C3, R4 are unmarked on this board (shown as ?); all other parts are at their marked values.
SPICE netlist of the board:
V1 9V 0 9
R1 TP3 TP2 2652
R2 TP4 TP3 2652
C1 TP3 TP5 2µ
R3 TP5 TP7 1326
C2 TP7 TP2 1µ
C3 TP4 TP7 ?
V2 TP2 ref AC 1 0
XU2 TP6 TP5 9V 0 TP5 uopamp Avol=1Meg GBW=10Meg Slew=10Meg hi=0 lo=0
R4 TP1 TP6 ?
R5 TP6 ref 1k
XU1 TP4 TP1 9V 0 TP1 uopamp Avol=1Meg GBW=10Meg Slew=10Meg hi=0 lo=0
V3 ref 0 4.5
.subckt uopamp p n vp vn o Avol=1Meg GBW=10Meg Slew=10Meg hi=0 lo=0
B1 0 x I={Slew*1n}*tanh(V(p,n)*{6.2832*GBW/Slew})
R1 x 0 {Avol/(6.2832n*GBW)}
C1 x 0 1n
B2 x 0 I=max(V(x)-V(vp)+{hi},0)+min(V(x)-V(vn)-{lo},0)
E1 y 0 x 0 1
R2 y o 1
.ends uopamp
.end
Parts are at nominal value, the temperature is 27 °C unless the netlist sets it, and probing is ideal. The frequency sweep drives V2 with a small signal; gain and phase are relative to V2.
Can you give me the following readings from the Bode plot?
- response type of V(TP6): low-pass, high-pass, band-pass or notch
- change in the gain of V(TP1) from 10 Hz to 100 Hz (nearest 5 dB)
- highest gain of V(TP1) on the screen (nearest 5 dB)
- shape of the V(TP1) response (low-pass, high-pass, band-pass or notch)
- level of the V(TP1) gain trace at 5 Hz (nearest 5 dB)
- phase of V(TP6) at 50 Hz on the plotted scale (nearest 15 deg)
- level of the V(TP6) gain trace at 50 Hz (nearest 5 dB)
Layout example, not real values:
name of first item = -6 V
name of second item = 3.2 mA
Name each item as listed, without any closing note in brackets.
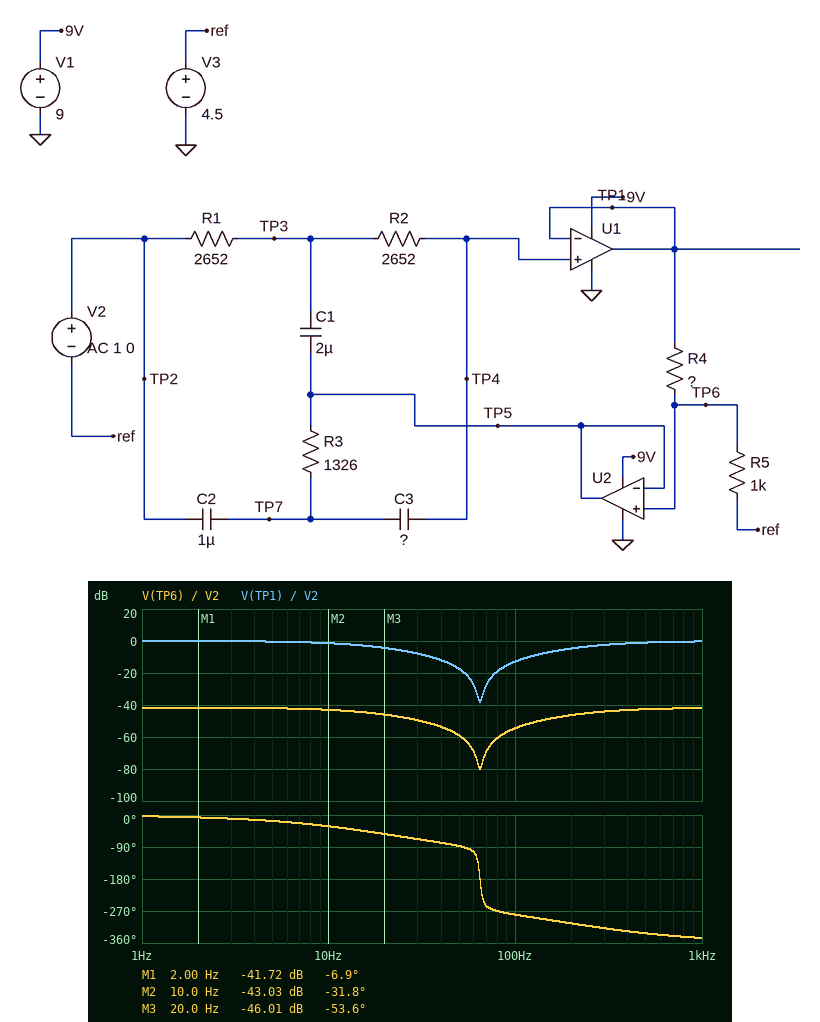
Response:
response type of V(TP6): low-pass, high-pass, band-pass or notch = notch
change in the gain of V(TP1) from 10 Hz to 100 Hz = -10 dB
highest gain of V(TP1) on the screen = 0 dB
shape of the V(TP1) response = notch
level of the V(TP1) gain trace at 5 Hz = 0 dB
phase of V(TP6) at 50 Hz on the plotted scale = -90 deg
level of the V(TP6) gain trace at 50 Hz = -60 dB
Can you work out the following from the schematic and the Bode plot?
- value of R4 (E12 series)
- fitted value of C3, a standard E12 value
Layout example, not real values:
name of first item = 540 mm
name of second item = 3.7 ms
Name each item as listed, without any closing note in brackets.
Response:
value of R4 = 120 kΩ
fitted value of C3, a standard E12 value = 820 nF
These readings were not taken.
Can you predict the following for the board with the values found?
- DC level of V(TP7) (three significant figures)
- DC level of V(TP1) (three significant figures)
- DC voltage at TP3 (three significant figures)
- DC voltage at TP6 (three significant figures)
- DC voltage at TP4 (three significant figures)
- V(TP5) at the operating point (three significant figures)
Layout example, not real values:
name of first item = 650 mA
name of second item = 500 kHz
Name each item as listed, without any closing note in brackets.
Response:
DC level of V(TP7) = 4.50 V
DC level of V(TP1) = 4.50 V
DC voltage at TP3 = 4.50 V
DC voltage at TP6 = 4.50 V
DC voltage at TP4 = 4.50 V
V(TP5) at the operating point = 4.50 V
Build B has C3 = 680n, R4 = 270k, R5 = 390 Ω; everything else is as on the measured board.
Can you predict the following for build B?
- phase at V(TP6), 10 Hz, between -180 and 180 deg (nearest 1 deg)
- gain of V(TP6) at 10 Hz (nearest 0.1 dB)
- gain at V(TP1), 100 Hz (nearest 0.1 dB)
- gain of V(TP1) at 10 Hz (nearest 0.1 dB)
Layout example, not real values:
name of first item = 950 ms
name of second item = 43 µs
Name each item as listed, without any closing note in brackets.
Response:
phase at V(TP6), 10 Hz, between -180 and 180 deg = -30 deg
gain of V(TP6) at 10 Hz = -58.0 dB
gain at V(TP1), 100 Hz = -14.2 dB
gain of V(TP1) at 10 Hz = -1.2 dB
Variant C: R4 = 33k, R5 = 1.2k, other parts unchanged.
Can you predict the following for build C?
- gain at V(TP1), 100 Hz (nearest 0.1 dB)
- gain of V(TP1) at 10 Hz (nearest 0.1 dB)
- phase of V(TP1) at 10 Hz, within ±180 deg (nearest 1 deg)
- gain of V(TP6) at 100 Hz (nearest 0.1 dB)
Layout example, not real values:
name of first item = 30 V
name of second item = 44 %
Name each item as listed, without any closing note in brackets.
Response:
gain at V(TP1), 100 Hz = -12.6 dB
gain of V(TP1) at 10 Hz = -1.3 dB
phase of V(TP1) at 10 Hz, within ±180 deg = -31 deg
gain of V(TP6) at 100 Hz = -41.7 dB
